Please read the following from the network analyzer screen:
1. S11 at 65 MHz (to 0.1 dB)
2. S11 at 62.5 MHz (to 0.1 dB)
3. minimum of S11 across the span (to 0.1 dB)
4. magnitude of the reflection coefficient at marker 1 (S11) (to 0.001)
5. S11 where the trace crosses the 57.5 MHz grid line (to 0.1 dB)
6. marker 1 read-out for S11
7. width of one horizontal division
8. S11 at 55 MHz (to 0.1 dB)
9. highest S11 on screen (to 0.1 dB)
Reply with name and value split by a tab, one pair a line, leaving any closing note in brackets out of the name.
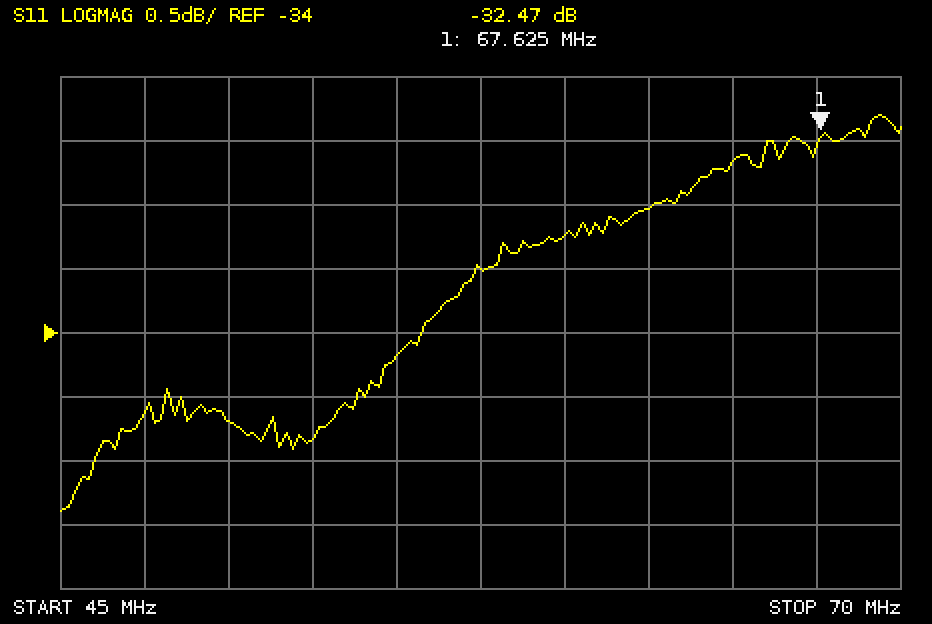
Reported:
S11 at 65 MHz	-32.7 dB
S11 at 62.5 MHz	-33.0 dB
minimum of S11 across the span	-35.4 dB
magnitude of the reflection coefficient at marker 1 (S11)	0.024
S11 where the trace crosses the 57.5 MHz grid line	-33.5 dB
marker 1 read-out for S11	-32.47 dB
width of one horizontal division	2.5 MHz
S11 at 55 MHz	-34.2 dB
highest S11 on screen	-32.3 dB
